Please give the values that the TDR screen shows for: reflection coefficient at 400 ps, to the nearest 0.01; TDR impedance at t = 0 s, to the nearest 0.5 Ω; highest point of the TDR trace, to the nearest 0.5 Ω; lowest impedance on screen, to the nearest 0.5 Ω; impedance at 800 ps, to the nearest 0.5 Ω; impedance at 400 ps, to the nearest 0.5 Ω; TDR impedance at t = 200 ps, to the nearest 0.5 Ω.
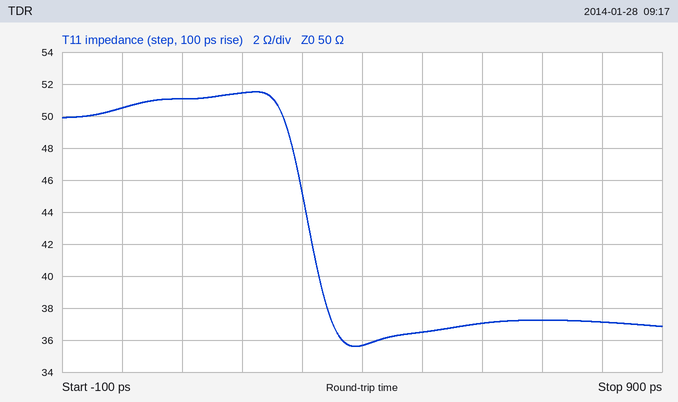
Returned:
-0.17
50.5 Ω
51.5 Ω
35.5 Ω
37.0 Ω
35.5 Ω
51.5 Ω
